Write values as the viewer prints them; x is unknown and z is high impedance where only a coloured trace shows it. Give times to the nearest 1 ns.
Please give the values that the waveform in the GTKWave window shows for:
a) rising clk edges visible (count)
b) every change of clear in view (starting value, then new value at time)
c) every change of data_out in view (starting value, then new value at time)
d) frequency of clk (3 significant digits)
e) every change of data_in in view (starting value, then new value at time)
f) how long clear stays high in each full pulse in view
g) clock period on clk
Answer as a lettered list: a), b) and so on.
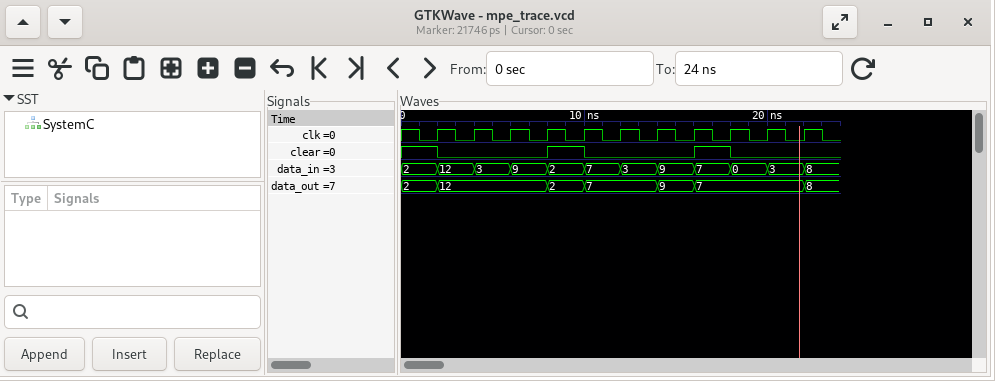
a) 11
b) 1, 0 at 2 ns, 1 at 8 ns, 0 at 10 ns, 1 at 16 ns, 0 at 18 ns
c) 2, 12 at 2 ns, 2 at 8 ns, 7 at 10 ns, 9 at 14 ns, 7 at 16 ns, 8 at 22 ns
d) 500 MHz
e) 2, 12 at 2 ns, 3 at 4 ns, 9 at 6 ns, 2 at 8 ns, 7 at 10 ns, 3 at 12 ns, 9 at 14 ns, 7 at 16 ns, 0 at 18 ns, 3 at 20 ns, 8 at 22 ns
f) 2 ns, 2 ns
g) 2 ns
